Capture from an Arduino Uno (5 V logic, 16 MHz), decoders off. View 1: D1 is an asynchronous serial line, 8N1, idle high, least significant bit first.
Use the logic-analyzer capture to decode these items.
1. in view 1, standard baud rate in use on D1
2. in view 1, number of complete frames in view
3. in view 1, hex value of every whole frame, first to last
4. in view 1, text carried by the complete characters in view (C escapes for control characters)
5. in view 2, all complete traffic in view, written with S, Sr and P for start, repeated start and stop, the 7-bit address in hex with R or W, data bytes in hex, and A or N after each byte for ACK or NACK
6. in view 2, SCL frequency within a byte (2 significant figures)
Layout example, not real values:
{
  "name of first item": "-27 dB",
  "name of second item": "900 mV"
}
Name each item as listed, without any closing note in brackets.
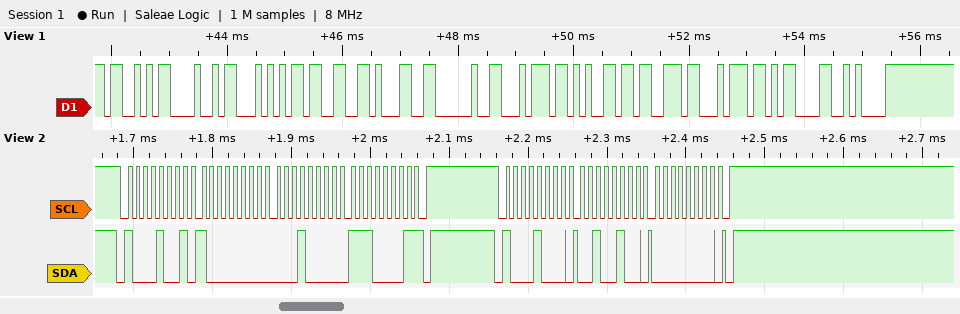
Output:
{
  "in view 1, standard baud rate in use on D1": "9600 baud",
  "in view 1, number of complete frames in view": "12",
  "in view 1, hex value of every whole frame, first to last": "53 48 54 33 31 20 74 65 73 74 0D 0A",
  "in view 1, text carried by the complete characters in view": "\"SHT31 test\\r\\n\"",
  "in view 2, all complete traffic in view, written with S, Sr and P for start, repeated start and stop, the 7-bit address in hex with R or W, data bytes in hex, and A or N after each byte for ACK or NACK": "S 44R A 80 A 10 A E1 N P S 44W A 24 A 00 A P",
  "in view 2, SCL frequency within a byte": "100 kHz"
}
